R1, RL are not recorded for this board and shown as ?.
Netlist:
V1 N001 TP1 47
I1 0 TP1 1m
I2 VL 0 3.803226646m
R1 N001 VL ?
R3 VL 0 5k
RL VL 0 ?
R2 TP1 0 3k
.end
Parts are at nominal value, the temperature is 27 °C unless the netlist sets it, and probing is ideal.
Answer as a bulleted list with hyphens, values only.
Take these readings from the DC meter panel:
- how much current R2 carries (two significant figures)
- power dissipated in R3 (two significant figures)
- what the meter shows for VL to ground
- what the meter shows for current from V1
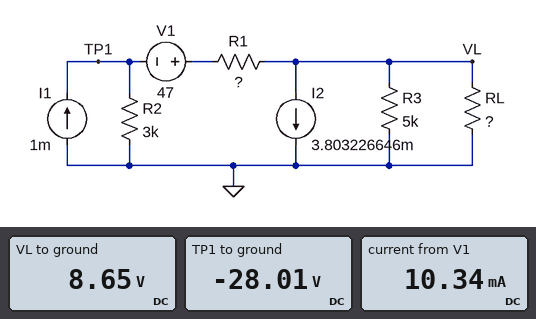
- 9.3 mA
- 15 mW
- 8.65 V
- 10.34 mA
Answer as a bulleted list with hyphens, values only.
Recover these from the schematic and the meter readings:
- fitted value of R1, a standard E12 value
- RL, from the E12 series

- 1 kΩ
- 1.8 kΩ
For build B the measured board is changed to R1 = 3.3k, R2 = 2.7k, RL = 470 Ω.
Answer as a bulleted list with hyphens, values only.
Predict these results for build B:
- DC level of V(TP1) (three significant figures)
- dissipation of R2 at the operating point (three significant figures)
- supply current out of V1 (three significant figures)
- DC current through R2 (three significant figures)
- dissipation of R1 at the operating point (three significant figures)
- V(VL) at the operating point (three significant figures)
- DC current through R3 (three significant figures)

- -18.9 V
- 132 mW
- 7.98 mA
- 6.98 mA
- 210 mW
- 1.80 V
- 359 µA
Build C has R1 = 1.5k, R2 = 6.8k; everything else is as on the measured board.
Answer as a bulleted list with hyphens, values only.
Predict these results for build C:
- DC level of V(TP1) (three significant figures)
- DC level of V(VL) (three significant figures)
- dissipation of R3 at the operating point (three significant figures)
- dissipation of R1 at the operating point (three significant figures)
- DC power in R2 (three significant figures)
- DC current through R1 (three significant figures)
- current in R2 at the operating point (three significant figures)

- -34.8 V
- 3.06 V
- 1.87 mW
- 56.1 mW
- 178 mW
- 6.11 mA
- 5.11 mA
